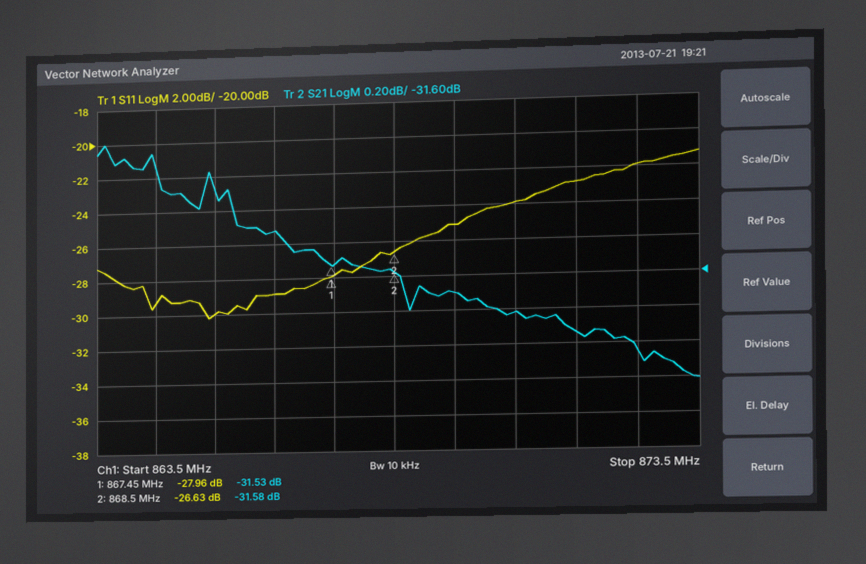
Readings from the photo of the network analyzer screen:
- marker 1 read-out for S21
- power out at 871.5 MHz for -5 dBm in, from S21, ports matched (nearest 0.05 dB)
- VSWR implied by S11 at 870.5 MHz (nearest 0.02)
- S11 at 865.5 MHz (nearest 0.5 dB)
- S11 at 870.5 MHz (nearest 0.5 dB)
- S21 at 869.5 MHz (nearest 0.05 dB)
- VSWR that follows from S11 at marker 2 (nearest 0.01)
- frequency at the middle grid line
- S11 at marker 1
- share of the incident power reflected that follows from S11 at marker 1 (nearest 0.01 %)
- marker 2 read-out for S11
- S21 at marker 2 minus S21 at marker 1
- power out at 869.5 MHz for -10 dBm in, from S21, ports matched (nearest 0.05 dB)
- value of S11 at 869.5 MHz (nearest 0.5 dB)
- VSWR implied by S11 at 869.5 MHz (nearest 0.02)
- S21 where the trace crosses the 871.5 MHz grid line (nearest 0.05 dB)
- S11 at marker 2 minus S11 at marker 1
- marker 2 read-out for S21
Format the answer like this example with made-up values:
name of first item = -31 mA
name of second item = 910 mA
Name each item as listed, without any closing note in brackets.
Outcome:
marker 1 read-out for S21 = -31.53 dB
power out at 871.5 MHz for -5 dBm in, from S21, ports matched = -36.95 dBm
VSWR implied by S11 at 870.5 MHz = 1.14
S11 at 865.5 MHz = -30.0 dB
S11 at 870.5 MHz = -24.0 dB
S21 at 869.5 MHz = -31.70 dB
VSWR that follows from S11 at marker 2 = 1.10
frequency at the middle grid line = 868.5 MHz
S11 at marker 1 = -27.96 dB
share of the incident power reflected that follows from S11 at marker 1 = 0.16 %
marker 2 read-out for S11 = -26.63 dB
S21 at marker 2 minus S21 at marker 1 = -0.05 dB
power out at 869.5 MHz for -10 dBm in, from S21, ports matched = -41.70 dBm
value of S11 at 869.5 MHz = -25.0 dB
VSWR implied by S11 at 869.5 MHz = 1.12
S21 where the trace crosses the 871.5 MHz grid line = -31.95 dB
S11 at marker 2 minus S11 at marker 1 = 1.33 dB
marker 2 read-out for S21 = -31.58 dB
